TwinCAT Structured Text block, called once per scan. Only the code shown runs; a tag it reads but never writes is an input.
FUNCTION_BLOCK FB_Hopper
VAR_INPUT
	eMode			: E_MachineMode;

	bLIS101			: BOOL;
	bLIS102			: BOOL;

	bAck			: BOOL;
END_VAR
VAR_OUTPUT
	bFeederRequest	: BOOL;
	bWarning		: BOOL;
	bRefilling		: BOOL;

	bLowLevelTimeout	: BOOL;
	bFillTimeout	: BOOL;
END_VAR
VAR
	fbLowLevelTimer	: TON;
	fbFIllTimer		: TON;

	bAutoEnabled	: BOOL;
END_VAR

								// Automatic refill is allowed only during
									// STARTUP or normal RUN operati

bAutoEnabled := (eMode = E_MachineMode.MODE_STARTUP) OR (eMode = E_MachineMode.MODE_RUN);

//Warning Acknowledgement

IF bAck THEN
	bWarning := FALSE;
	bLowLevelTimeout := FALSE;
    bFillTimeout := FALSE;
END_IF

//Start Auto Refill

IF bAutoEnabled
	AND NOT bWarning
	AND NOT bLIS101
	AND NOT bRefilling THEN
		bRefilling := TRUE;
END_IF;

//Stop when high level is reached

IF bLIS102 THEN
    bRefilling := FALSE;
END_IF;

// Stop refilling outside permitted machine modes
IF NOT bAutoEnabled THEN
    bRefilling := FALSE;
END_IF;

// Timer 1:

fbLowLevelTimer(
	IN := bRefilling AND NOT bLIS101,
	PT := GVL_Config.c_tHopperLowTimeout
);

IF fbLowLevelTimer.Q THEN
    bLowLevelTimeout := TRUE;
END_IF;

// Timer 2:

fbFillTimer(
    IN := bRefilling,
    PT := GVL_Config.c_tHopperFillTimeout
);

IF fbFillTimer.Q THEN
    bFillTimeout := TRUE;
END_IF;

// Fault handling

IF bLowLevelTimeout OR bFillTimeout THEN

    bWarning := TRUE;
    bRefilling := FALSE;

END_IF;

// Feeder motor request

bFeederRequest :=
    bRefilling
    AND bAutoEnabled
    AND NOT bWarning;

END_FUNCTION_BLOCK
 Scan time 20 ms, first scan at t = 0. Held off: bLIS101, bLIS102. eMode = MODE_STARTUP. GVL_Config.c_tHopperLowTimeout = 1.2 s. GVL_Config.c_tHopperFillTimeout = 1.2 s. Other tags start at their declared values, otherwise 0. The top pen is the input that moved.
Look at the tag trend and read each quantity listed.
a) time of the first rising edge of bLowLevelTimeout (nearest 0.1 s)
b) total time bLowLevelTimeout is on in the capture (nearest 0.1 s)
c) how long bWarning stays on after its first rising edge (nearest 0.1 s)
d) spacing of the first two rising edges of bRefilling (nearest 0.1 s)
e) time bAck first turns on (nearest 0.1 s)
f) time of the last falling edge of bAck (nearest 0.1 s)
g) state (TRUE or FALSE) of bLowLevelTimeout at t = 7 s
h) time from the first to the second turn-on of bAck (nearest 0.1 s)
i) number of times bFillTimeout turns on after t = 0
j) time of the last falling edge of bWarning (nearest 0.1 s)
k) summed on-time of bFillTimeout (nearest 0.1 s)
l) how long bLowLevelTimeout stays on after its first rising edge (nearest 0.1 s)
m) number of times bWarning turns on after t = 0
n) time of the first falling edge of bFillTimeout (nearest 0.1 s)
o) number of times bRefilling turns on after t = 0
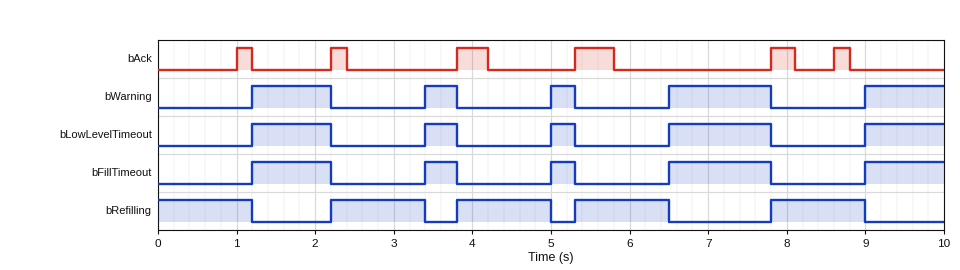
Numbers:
1.2 s
4.0 s
1.0 s
1.6 s
1.0 s
8.8 s
TRUE
1.2 s
5
7.8 s
4.0 s
1.0 s
5
2.2 s
4
